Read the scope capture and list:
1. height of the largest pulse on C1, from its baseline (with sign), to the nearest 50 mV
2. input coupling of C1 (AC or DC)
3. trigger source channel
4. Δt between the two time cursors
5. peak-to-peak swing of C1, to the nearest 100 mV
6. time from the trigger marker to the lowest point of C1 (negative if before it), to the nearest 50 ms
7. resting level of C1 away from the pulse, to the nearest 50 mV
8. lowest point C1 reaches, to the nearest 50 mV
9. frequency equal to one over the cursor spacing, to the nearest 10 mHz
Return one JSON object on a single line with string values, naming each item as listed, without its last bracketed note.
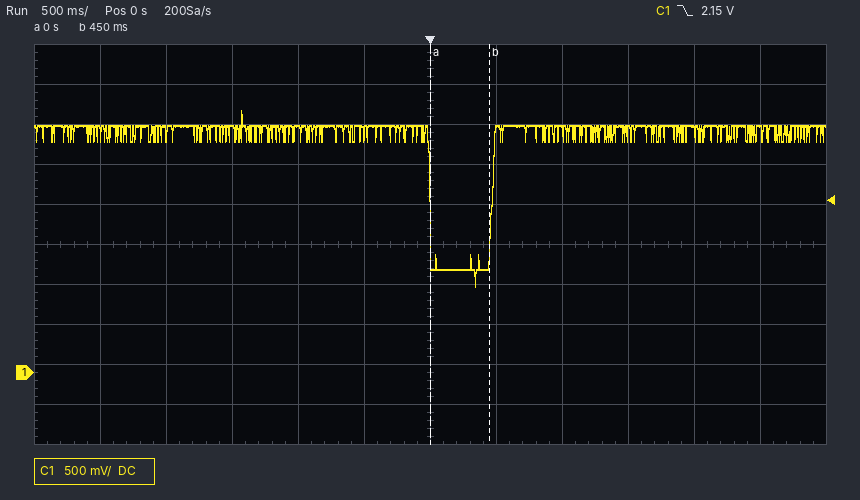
{"height of the largest pulse on C1, from its baseline (with sign), to the nearest 50 mV": "-2.00 V", "input coupling of C1": "DC", "trigger source channel": "C1", "Δt between the two time cursors": "450 ms", "peak-to-peak swing of C1, to the nearest 100 mV": "2.20 V", "time from the trigger marker to the lowest point of C1 (negative if before it), to the nearest 50 ms": "+350 ms", "resting level of C1 away from the pulse, to the nearest 50 mV": "3.10 V", "lowest point C1 reaches, to the nearest 50 mV": "1.10 V", "frequency equal to one over the cursor spacing, to the nearest 10 mHz": "2.22 Hz"}
